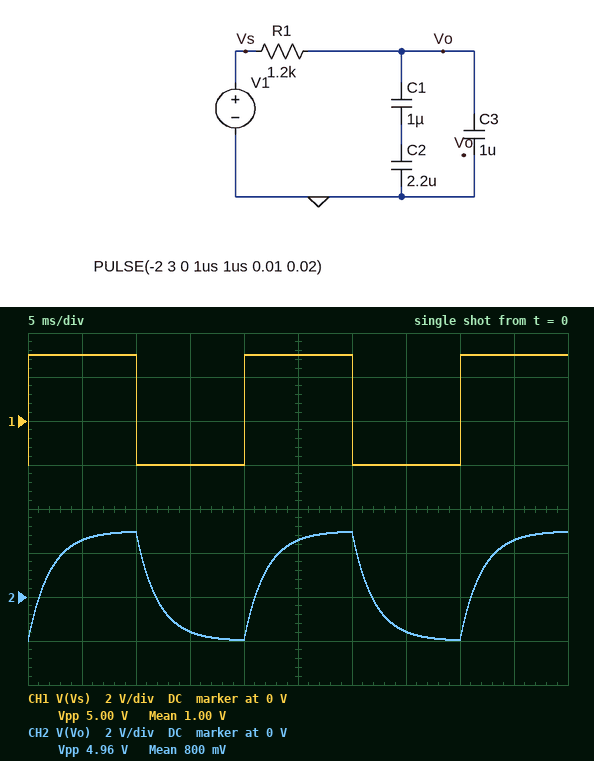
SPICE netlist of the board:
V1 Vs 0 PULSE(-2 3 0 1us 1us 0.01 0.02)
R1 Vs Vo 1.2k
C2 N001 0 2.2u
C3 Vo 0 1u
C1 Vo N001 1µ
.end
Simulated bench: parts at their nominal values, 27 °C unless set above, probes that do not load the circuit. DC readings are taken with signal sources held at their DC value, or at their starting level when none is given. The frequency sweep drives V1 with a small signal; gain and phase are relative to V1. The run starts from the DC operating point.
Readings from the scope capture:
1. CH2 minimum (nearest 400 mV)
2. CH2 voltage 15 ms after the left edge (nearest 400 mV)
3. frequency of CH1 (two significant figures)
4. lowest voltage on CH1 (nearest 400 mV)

-2.0 V
-1.6 V
50 Hz
-2.0 V
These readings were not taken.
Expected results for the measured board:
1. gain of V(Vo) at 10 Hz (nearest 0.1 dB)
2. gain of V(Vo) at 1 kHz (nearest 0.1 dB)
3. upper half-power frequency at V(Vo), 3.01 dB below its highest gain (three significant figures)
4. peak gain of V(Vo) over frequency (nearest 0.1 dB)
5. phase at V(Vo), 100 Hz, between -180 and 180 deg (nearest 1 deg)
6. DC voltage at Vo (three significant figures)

-0.1 dB
-22.1 dB
78.6 Hz
0 dB
-52 deg
-2.00 V
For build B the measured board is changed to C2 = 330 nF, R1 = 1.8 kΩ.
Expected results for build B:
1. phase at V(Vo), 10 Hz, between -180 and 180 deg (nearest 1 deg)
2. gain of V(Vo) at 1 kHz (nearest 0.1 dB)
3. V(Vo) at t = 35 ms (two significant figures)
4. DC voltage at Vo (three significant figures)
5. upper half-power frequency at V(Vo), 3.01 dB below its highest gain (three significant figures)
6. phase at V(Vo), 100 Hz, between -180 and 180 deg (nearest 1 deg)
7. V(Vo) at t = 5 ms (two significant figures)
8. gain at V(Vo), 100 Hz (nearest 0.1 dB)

-8 deg
-23.0 dB
-1.5 V
-2.00 V
70.8 Hz
-55 deg
2.5 V
-4.8 dB
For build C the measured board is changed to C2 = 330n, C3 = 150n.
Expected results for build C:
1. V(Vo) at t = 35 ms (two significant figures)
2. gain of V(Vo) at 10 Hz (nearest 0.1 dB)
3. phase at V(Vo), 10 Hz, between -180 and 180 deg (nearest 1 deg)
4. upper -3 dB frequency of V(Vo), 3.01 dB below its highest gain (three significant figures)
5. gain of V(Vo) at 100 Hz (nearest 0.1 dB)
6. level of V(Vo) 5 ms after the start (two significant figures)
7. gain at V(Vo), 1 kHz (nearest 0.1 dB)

-2.0 V
0 dB
-2 deg
333 Hz
-0.4 dB
3.0 V
-10.0 dB
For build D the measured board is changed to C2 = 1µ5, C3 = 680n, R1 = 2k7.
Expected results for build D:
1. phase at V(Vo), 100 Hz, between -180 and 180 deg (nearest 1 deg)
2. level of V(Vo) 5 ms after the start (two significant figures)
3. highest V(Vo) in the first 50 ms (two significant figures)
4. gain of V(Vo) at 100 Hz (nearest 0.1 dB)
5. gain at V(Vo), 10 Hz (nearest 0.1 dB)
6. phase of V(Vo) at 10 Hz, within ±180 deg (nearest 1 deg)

-65 deg
1.8 V
2.7 V
-7.6 dB
-0.2 dB
-12 deg
